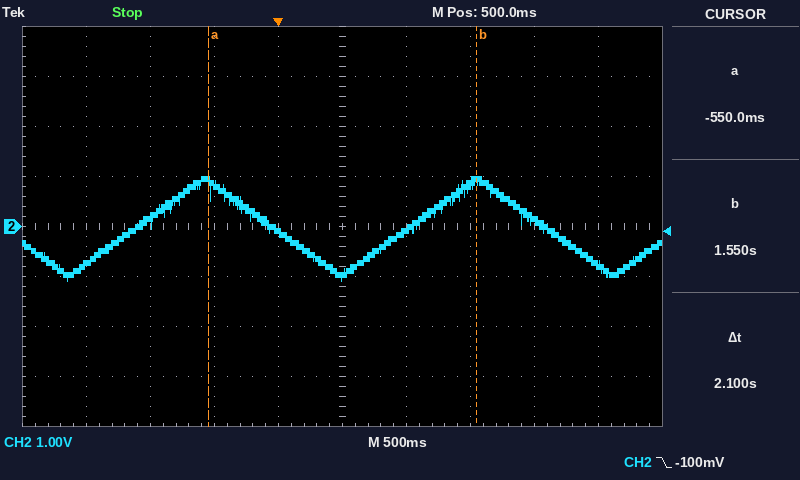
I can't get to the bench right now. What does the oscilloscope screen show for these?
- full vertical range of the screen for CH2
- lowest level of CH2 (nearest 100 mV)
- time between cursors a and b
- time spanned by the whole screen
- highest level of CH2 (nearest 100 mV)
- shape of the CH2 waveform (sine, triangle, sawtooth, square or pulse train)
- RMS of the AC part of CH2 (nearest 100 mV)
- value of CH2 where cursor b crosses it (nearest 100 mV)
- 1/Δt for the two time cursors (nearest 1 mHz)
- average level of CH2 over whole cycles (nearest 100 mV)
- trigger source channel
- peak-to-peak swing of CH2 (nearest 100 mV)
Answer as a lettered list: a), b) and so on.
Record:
a) 8 V
b) -1.1 V
c) 2.1 s
d) 5 s
e) 1.0 V
f) triangle
g) 600 mV
h) 900 mV
i) 476 mHz
j) 0.0 V
k) CH2
l) 2.1 V
